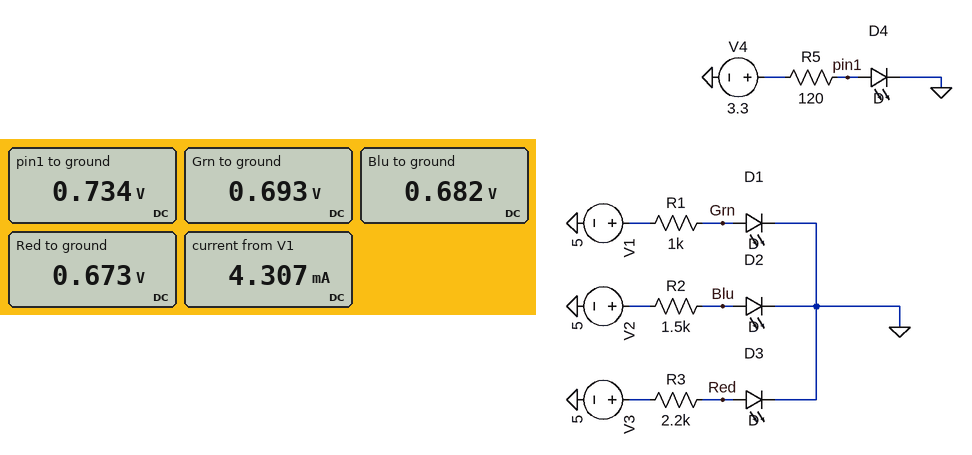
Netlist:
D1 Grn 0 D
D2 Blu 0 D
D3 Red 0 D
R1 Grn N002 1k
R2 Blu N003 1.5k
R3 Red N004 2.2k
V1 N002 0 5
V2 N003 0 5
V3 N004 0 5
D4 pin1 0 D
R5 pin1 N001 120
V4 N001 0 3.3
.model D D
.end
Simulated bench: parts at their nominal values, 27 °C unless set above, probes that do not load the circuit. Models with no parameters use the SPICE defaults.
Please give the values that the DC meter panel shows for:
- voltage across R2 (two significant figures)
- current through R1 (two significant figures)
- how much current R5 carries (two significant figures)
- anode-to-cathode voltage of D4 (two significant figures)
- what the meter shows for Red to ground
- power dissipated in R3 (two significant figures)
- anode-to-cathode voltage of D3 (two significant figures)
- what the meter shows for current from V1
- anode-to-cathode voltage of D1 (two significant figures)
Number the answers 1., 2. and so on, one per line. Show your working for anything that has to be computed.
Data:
1. 5 V - 682 mV = 4.3 V
2. (5 V - 693 mV) / 1 kΩ = 4.3 mA
3. (3.3 V - 734 mV) / 120 Ω = 21 mA
4. 734 mV = 730 mV
5. 0.673 V
6. (5 V - 673 mV)^2 / 2.2 kΩ = 8.5 mW
7. 673 mV = 670 mV
8. 4.307 mA
9. 693 mV = 690 mV
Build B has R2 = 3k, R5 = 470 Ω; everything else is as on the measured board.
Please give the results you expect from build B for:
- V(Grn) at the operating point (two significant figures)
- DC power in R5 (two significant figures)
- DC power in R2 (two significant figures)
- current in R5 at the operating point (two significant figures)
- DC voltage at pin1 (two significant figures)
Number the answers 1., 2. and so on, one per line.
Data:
1. 690 mV
2. 14 mW
3. 6.3 mW
4. 5.5 mA
5. 700 mV
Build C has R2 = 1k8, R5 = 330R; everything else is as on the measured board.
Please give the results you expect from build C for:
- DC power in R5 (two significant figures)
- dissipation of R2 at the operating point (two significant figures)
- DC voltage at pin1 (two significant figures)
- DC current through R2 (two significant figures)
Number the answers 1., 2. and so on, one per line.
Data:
1. 20 mW
2. 10 mW
3. 710 mV
4. 2.4 mA
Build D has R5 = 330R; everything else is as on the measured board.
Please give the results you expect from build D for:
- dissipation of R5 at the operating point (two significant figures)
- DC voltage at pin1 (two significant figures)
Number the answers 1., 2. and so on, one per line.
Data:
1. 20 mW
2. 710 mV
